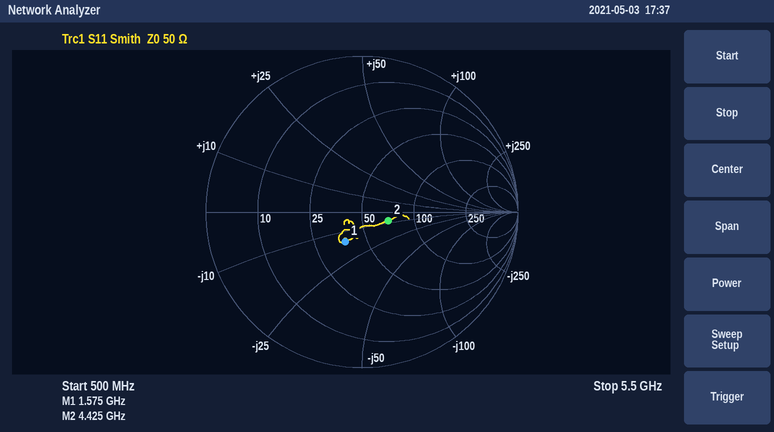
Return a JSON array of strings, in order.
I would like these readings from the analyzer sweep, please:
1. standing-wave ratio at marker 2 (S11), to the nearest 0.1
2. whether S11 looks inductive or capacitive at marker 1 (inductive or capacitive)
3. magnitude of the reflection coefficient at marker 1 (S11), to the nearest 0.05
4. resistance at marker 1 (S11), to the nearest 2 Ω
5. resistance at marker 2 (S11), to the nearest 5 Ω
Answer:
["1.4", "capacitive", "0.20", "38 Ω", "70 Ω"]
